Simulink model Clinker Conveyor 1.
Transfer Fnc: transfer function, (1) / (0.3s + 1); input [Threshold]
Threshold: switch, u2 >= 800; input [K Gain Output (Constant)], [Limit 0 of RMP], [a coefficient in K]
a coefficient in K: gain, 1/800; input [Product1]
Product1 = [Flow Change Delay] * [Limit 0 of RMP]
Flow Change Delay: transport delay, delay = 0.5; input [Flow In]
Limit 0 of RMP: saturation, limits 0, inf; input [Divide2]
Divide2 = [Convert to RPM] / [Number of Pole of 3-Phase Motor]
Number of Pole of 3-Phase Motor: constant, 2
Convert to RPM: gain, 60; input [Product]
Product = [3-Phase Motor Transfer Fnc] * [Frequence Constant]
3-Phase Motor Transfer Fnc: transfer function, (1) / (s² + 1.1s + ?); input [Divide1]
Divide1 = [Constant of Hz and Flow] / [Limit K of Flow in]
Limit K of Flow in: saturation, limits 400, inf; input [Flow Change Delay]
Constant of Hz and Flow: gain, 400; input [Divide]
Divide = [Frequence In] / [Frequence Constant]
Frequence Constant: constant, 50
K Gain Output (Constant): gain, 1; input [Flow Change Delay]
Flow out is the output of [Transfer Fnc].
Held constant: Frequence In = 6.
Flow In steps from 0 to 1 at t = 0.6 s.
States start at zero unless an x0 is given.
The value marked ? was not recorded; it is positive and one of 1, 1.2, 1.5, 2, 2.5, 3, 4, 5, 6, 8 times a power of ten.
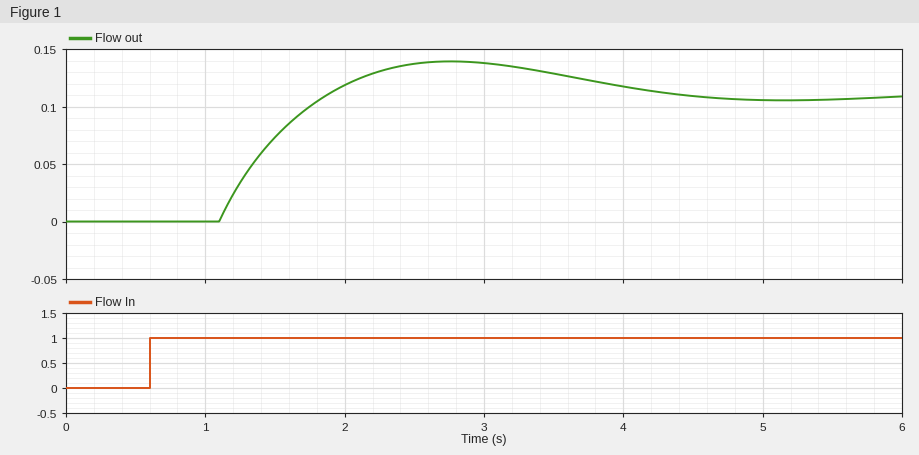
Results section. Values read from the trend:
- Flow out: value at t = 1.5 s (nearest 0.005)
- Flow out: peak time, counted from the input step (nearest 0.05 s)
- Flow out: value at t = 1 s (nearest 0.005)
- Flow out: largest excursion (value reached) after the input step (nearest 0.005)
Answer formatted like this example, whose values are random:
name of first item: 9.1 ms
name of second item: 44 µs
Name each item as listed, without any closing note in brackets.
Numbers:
Flow out: value at t = 1.5 s: 0.075
Flow out: peak time, counted from the input step: 2.15 s
Flow out: value at t = 1 s: 0.000
Flow out: largest excursion (value reached) after the input step: 0.140
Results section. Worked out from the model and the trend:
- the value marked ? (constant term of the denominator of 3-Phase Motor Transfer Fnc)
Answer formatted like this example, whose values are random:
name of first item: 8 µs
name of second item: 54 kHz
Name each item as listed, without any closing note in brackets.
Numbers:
the value marked ?: 2
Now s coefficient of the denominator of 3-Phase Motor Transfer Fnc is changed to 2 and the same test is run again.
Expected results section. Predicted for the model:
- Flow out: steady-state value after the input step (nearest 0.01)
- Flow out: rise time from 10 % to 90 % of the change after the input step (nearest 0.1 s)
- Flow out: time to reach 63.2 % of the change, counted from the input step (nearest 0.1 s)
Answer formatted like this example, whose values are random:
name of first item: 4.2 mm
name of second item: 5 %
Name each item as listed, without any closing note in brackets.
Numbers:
Flow out: steady-state value after the input step: 0.11
Flow out: rise time from 10 % to 90 % of the change after the input step: 1.1 s
Flow out: time to reach 63.2 % of the change, counted from the input step: 1.1 s
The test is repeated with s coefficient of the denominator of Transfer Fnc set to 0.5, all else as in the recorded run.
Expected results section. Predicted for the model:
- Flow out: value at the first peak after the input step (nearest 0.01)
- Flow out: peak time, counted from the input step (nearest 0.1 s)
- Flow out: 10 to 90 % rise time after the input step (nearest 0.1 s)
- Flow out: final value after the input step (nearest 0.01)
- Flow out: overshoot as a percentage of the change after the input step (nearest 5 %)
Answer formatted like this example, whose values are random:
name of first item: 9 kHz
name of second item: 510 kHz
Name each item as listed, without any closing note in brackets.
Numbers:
Flow out: value at the first peak after the input step: 0.13
Flow out: peak time, counted from the input step: 2.4 s
Flow out: 10 to 90 % rise time after the input step: 0.8 s
Flow out: final value after the input step: 0.11
Flow out: overshoot as a percentage of the change after the input step: 20 %
